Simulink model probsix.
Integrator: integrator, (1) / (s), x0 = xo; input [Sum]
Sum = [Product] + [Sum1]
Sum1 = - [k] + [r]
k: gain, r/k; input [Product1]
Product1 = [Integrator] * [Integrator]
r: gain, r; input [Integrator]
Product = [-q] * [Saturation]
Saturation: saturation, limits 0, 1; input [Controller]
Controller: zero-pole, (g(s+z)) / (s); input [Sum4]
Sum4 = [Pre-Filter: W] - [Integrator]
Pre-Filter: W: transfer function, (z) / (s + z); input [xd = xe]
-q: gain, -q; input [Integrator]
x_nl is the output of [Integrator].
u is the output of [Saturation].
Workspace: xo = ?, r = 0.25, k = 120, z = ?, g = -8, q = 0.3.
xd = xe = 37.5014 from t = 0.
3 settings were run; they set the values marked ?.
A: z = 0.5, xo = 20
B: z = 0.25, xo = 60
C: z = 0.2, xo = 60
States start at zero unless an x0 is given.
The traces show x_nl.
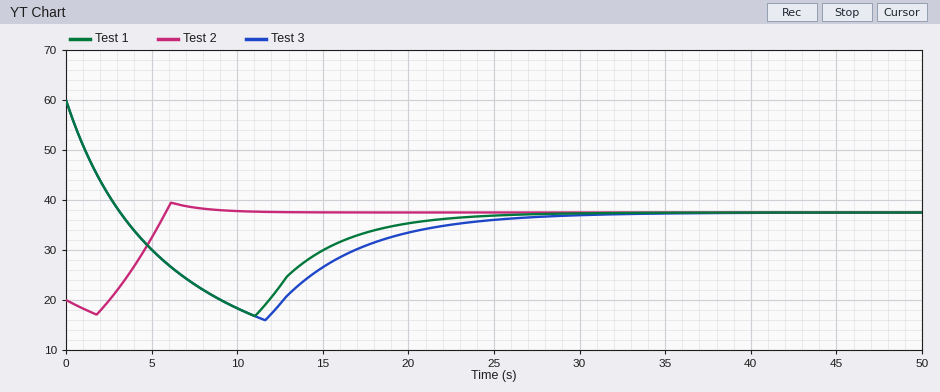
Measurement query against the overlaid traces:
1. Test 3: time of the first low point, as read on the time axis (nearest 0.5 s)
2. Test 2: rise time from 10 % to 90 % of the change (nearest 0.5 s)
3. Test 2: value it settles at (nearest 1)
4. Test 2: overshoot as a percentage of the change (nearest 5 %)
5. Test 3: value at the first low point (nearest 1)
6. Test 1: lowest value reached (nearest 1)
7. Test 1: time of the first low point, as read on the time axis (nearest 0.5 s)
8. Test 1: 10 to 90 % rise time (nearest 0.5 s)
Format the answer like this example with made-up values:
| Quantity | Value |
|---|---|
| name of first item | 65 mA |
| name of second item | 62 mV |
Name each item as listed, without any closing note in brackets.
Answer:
| Quantity | Value |
|---|---|
| Test 3: time of the first low point, as read on the time axis | 11.5 s |
| Test 2: rise time from 10 % to 90 % of the change | 2.5 s |
| Test 2: value it settles at | 38 |
| Test 2: overshoot as a percentage of the change | 10 % |
| Test 3: value at the first low point | 16 |
| Test 1: lowest value reached | 17 |
| Test 1: time of the first low point, as read on the time axis | 11.0 s |
| Test 1: 10 to 90 % rise time | 2.5 s |
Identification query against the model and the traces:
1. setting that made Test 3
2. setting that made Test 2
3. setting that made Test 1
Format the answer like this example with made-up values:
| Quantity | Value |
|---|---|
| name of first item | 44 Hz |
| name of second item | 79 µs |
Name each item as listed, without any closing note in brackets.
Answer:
| Quantity | Value |
|---|---|
| setting that made Test 3 | C |
| setting that made Test 2 | A |
| setting that made Test 1 | B |
